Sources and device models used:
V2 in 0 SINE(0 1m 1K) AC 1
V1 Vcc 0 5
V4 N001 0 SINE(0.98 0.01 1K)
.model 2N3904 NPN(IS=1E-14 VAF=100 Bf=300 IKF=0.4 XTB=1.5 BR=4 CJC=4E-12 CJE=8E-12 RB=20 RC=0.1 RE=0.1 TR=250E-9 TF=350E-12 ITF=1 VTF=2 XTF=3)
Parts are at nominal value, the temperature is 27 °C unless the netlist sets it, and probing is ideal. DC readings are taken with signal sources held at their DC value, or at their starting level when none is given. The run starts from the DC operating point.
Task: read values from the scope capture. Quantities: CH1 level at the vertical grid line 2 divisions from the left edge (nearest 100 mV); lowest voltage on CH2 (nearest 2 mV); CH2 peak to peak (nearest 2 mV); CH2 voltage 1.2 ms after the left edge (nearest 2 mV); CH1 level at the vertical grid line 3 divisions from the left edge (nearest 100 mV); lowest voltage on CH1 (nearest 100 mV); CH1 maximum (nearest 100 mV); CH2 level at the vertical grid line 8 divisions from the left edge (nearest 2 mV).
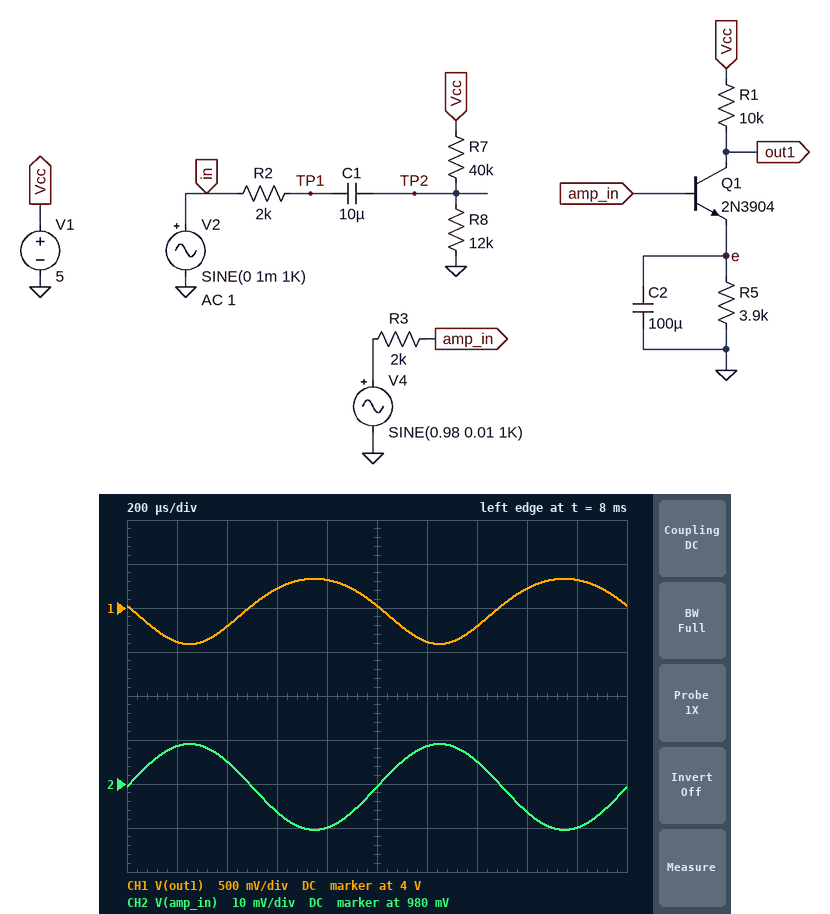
3.8 V
970 mV
20 mV
988 mV
4.2 V
3.6 V
4.3 V
974 mV
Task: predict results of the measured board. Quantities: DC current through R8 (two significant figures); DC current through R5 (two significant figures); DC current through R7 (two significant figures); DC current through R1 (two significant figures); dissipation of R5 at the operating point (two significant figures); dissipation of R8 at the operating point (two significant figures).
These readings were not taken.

96 µA
99 µA
96 µA
98 µA
38 µW
110 µW
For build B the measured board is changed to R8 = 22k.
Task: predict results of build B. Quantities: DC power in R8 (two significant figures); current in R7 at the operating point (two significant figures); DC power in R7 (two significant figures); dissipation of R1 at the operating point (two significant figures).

140 µW
81 µA
260 µW
97 µW
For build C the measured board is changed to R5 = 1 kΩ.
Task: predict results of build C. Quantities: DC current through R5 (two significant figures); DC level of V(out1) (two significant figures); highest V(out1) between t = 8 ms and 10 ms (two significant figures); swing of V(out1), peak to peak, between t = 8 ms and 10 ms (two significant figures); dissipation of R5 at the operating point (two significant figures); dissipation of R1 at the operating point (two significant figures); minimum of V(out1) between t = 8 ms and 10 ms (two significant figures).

350 µA
1.5 V
2.6 V
2.1 V
120 µW
1.2 mW
480 mV
